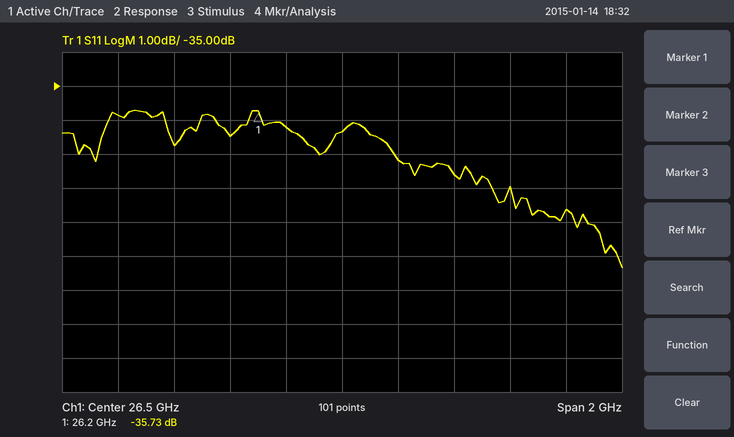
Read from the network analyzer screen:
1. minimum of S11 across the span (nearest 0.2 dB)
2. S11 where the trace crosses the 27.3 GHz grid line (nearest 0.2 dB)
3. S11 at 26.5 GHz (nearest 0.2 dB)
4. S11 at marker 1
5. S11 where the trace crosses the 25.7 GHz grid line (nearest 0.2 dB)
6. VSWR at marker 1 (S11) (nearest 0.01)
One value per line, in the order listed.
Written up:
-40.4 dB
-38.6 dB
-36.4 dB
-35.73 dB
-35.8 dB
1.03
